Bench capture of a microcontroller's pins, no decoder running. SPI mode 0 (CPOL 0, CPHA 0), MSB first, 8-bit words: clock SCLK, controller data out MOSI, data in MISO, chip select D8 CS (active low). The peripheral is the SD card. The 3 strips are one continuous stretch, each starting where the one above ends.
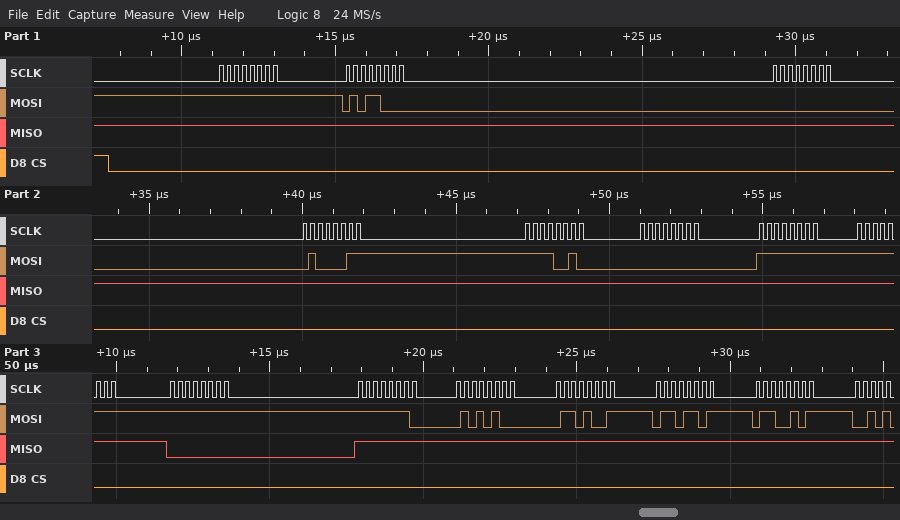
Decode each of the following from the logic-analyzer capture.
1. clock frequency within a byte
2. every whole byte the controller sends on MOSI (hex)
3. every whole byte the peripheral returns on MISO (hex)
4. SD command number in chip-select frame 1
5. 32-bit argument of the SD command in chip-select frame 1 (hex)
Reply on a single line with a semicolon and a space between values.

4 MHz; FF 58 00 43 F2 00 FF FF FF FE 54 69 6D 65; FF FF FF FF FF FF FF FF 00 FF FF FF FF FF; CMD24; 0x0043F200
